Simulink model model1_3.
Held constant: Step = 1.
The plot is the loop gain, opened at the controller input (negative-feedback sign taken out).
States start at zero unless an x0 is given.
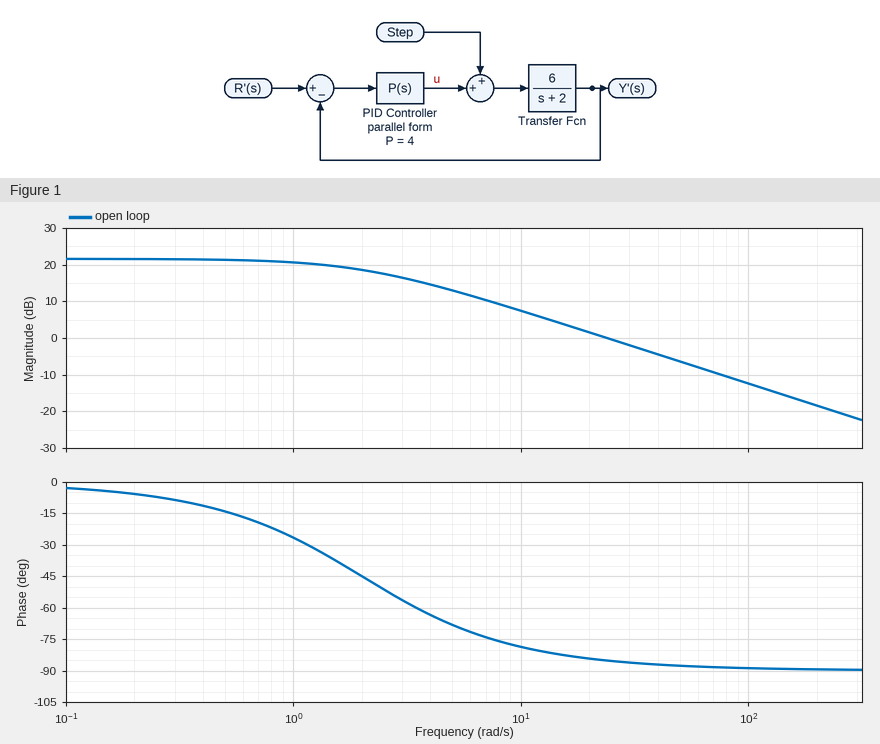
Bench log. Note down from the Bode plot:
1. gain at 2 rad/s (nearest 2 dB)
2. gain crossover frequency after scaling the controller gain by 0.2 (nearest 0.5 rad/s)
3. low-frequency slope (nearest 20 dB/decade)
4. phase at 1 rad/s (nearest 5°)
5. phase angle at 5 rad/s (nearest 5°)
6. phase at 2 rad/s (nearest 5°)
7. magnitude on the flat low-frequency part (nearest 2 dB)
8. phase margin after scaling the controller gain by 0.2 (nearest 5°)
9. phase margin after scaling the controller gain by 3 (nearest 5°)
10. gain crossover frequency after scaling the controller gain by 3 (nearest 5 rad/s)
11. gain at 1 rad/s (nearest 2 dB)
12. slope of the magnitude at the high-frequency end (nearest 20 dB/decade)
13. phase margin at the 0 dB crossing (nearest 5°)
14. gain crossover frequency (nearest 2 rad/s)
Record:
18 dB
4.5 rad/s
0 dB/decade
-25°
-70°
-45°
22 dB
115°
90°
70 rad/s
20 dB
-20 dB/decade
95°
24 rad/s
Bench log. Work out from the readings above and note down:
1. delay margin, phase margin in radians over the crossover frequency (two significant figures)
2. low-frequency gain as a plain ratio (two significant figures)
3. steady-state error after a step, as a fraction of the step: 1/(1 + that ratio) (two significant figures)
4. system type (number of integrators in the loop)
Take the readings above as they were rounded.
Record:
0.069 s
13
0.071
0
